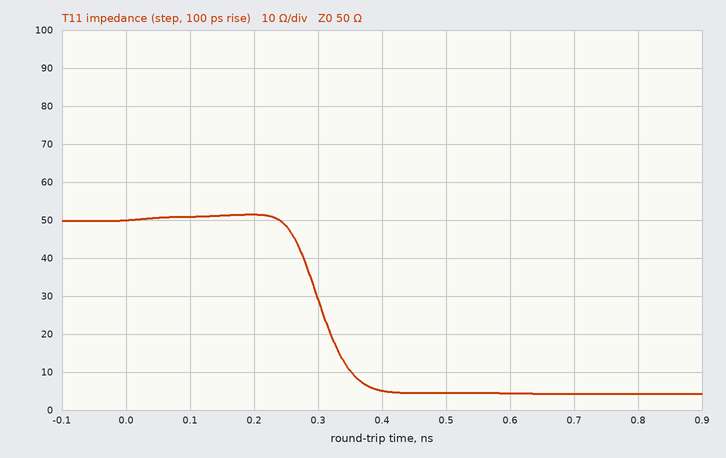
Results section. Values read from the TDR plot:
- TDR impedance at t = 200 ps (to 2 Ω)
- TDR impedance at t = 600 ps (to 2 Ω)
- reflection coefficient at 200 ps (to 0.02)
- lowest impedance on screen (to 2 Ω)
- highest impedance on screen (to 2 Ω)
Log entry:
52 Ω
4 Ω
+0.02
4 Ω
52 Ω
